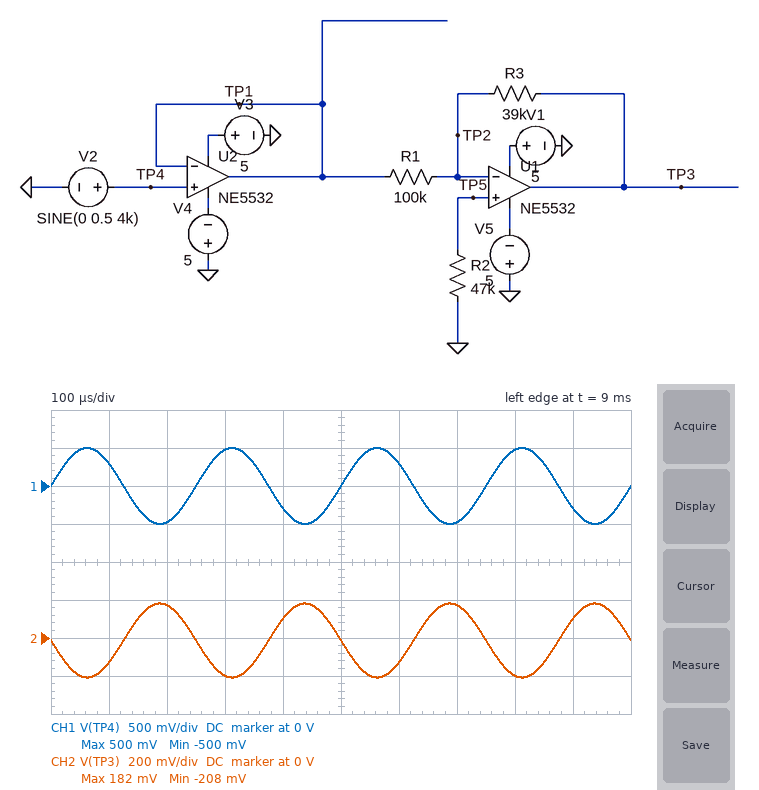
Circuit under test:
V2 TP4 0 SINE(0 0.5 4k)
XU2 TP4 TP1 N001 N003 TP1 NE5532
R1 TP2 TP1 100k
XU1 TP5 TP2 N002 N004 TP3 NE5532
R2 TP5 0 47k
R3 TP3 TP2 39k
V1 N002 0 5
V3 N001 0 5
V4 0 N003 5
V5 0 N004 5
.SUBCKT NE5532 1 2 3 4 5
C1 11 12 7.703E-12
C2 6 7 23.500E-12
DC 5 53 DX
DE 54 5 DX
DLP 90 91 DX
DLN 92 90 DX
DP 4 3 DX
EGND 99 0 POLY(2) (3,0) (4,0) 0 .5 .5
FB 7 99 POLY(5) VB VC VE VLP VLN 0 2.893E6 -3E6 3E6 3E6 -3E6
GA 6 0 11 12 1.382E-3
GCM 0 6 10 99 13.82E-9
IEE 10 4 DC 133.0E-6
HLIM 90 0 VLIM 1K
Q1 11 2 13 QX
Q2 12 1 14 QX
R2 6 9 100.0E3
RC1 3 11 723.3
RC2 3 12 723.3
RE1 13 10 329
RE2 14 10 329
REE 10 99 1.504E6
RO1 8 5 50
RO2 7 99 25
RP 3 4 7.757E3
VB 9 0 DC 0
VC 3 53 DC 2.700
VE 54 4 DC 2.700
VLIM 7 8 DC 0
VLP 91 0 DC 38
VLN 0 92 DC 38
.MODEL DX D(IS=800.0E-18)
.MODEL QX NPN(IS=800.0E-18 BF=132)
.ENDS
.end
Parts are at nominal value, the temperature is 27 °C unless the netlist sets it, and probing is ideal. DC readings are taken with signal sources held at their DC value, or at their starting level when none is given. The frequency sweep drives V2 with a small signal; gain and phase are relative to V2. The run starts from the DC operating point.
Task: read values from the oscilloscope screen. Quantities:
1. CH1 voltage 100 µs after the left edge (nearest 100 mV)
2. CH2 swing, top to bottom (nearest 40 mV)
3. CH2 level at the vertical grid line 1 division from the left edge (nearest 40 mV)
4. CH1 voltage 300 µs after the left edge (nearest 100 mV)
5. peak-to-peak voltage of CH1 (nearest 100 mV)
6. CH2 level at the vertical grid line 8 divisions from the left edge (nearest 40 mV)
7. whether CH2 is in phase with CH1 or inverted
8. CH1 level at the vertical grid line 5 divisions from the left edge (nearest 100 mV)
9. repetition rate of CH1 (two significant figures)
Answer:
300 mV
400 mV
-120 mV
500 mV
1.0 V
-200 mV
inverted
0 V
4.0 kHz
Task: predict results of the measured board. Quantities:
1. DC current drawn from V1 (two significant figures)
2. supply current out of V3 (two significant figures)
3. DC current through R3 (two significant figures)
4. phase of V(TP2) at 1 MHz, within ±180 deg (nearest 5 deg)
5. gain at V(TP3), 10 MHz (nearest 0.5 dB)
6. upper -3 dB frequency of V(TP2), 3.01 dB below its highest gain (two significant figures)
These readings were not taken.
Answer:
1.4 mA
1.4 mA
260 nA
75 deg
-15.5 dB
13 MHz
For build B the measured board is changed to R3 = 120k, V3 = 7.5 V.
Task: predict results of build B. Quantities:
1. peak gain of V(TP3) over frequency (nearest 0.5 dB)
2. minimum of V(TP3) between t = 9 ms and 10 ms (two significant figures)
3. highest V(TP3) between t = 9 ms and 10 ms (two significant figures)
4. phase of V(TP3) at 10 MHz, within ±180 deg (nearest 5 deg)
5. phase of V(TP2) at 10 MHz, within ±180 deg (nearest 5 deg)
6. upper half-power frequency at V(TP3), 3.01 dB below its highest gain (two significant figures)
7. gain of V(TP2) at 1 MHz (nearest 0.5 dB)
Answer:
1.5 dB
-590 mV
610 mV
-10 deg
-65 deg
3.5 MHz
-16.0 dB
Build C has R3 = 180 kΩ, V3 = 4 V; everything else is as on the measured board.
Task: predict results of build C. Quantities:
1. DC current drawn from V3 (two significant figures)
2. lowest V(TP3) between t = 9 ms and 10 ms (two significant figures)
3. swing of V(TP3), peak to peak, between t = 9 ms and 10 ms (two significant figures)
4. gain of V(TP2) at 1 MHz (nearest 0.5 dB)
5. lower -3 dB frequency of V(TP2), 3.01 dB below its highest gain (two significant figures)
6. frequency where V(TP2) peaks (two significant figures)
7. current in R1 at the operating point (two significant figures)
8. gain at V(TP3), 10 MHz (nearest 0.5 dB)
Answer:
1.3 mA
-880 mV
1.8 V
-13.0 dB
2.2 MHz
6.6 MHz
230 nA
-10.0 dB
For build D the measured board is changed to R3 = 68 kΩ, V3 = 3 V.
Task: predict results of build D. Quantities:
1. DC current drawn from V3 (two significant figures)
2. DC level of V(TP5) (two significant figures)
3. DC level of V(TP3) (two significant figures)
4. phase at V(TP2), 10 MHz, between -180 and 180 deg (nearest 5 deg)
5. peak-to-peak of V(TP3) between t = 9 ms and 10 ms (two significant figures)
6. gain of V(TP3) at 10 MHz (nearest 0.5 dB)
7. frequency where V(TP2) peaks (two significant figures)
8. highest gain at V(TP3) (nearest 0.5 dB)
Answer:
1.2 mA
-23 mV
-5.4 mV
-60 deg
680 mV
-13.0 dB
7.7 MHz
-3.5 dB
